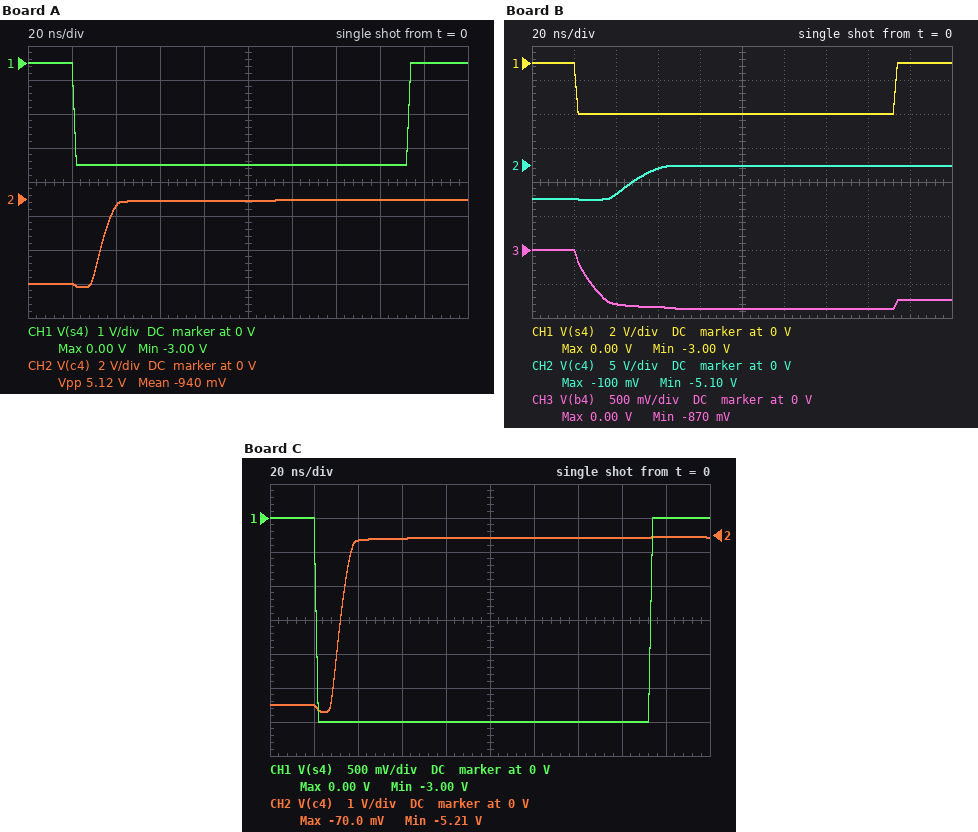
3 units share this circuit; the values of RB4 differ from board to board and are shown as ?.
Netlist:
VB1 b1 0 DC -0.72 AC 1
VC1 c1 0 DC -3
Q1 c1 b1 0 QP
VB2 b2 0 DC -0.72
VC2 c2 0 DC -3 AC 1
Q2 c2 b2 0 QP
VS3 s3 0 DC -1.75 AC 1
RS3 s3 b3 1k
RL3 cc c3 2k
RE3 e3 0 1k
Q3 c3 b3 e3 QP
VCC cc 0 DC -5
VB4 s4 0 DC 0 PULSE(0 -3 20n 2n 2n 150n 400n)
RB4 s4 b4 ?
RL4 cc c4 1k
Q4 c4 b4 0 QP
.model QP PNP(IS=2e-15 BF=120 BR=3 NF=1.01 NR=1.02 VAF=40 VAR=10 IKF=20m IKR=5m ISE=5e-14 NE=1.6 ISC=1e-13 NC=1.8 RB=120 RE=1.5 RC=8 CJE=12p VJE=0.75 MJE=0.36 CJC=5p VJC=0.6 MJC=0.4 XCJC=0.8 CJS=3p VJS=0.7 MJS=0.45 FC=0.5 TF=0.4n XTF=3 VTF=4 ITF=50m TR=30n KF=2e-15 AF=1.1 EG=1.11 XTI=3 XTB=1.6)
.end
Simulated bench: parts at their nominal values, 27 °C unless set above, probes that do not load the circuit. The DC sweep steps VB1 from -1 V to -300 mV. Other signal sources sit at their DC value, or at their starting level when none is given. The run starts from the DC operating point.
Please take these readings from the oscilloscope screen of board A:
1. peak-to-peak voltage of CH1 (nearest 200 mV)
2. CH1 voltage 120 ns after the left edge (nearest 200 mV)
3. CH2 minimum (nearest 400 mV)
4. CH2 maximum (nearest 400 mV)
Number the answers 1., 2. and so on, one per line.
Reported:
1. 3.0 V
2. -3.0 V
3. -5.2 V
4. 0 V
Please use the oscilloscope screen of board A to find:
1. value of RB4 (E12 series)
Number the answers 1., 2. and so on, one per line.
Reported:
1. 1.2 kΩ
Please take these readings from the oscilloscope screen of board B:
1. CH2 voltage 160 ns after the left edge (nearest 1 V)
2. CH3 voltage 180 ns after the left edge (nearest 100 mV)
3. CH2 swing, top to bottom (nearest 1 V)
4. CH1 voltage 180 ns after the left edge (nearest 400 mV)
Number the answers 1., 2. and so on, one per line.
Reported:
1. 0 V
2. -700 mV
3. 5 V
4. 0 V
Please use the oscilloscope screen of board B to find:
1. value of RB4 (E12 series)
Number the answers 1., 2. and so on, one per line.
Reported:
1. 2.7 kΩ
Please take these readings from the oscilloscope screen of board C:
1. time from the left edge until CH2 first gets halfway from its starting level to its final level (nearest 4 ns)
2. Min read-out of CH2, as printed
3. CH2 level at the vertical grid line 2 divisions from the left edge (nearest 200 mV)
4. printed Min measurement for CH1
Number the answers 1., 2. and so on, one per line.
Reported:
1. 32 ns
2. -5.21 V
3. -200 mV
4. -3.00 V
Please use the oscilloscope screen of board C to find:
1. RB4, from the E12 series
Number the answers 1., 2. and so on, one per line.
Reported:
1. 1 kΩ
